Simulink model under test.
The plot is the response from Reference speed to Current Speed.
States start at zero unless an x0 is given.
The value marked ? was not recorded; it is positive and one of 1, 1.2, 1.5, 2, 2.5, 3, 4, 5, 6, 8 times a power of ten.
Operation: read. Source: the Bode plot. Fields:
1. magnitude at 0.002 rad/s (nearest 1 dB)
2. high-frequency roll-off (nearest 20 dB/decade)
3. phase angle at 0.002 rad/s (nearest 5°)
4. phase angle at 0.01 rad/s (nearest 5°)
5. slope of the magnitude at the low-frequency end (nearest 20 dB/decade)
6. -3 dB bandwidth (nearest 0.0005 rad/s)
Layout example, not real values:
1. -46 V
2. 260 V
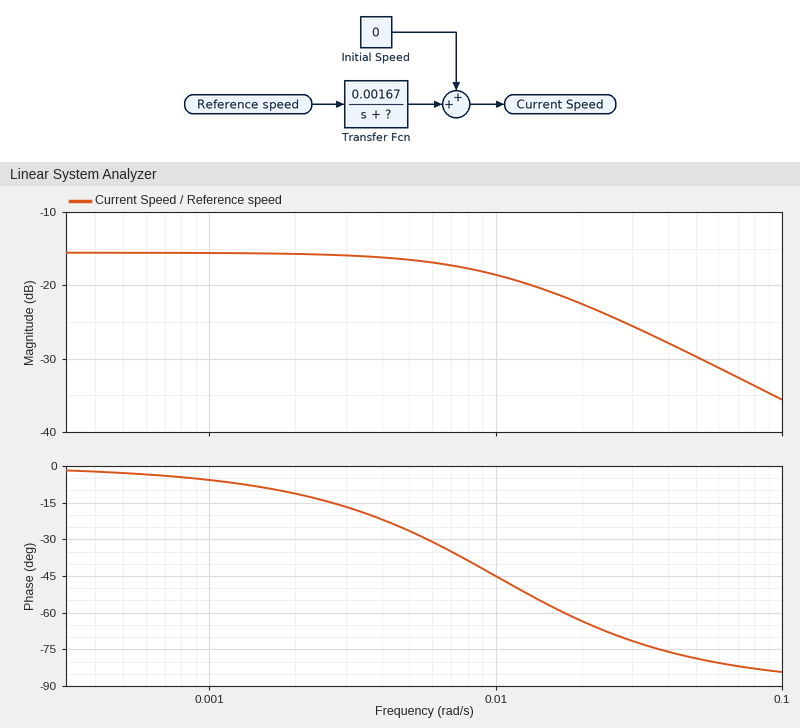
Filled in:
1. -16 dB
2. -20 dB/decade
3. -10°
4. -45°
5. 0 dB/decade
6. 0.0100 rad/s
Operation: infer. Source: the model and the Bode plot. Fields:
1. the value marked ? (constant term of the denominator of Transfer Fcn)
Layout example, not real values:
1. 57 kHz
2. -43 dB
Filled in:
1. 0.01
